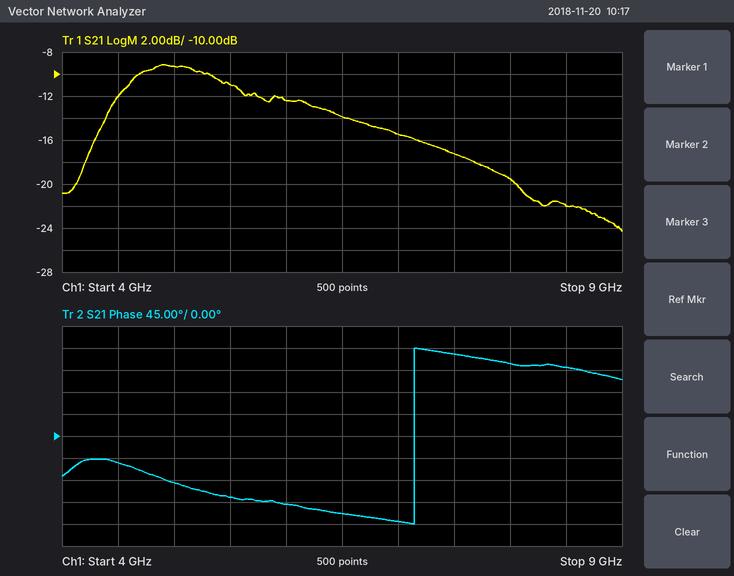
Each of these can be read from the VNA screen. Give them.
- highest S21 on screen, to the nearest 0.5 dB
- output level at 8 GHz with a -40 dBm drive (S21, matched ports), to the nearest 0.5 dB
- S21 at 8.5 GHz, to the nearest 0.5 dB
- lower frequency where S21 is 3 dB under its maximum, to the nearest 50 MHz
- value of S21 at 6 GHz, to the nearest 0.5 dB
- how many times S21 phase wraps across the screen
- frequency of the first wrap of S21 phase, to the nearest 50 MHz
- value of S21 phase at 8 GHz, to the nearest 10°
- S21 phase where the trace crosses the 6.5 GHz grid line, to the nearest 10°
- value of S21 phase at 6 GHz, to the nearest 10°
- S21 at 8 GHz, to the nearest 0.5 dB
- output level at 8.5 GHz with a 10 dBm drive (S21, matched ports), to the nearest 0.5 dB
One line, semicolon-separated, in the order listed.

-9.0 dB; -59.5 dBm; -22.0 dB; 4.50 GHz; -12.5 dB; 1; 7.15 GHz; 150°; -160°; -140°; -19.5 dB; -12.0 dBm
